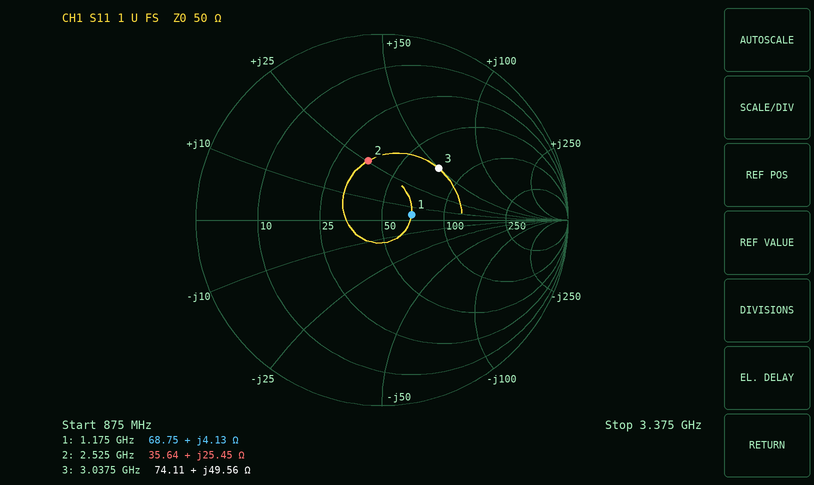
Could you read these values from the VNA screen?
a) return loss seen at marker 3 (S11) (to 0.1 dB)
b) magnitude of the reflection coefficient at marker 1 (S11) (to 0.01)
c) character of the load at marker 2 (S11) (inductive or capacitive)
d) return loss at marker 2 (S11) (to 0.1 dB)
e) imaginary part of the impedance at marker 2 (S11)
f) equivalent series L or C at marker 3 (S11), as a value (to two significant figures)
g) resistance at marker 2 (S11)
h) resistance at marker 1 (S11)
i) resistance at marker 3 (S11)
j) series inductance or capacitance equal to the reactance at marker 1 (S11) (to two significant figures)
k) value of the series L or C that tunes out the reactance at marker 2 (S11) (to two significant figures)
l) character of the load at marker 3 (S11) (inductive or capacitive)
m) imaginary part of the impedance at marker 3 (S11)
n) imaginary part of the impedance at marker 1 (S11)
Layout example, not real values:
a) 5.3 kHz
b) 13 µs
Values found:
a) 7.7 dB
b) 0.16
c) inductive
d) 9.7 dB
e) +25.45 Ω
f) 2.6 nH
g) 35.64 Ω
h) 68.75 Ω
i) 74.11 Ω
j) 560 pH
k) 2.5 pF
l) inductive
m) +49.56 Ω
n) +4.13 Ω
